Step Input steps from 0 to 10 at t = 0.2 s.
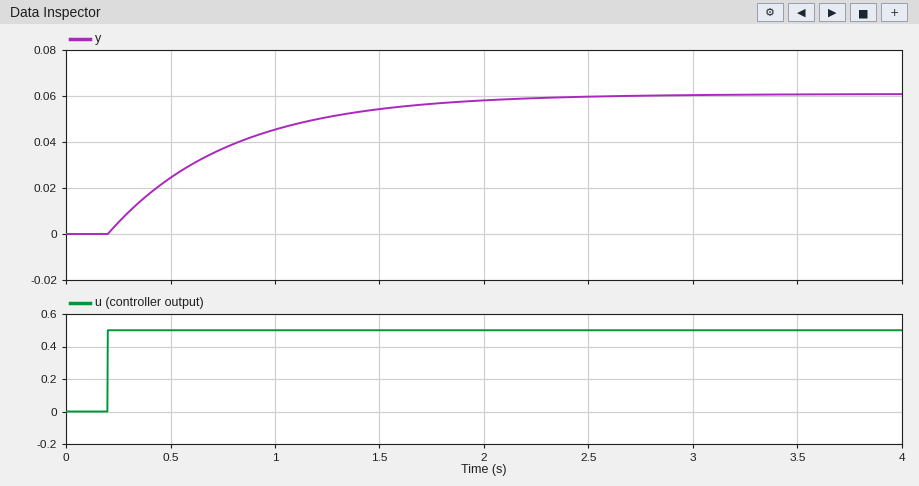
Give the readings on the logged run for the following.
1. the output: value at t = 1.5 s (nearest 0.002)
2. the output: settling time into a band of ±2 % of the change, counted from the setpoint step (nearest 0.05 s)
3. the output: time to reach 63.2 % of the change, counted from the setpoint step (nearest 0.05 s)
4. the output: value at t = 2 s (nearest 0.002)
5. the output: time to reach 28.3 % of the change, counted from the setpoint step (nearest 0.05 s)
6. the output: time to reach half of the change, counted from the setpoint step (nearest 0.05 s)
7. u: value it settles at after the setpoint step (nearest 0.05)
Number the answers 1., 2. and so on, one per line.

1. 0.054
2. 2.30 s
3. 0.60 s
4. 0.058
5. 0.20 s
6. 0.40 s
7. 0.50
